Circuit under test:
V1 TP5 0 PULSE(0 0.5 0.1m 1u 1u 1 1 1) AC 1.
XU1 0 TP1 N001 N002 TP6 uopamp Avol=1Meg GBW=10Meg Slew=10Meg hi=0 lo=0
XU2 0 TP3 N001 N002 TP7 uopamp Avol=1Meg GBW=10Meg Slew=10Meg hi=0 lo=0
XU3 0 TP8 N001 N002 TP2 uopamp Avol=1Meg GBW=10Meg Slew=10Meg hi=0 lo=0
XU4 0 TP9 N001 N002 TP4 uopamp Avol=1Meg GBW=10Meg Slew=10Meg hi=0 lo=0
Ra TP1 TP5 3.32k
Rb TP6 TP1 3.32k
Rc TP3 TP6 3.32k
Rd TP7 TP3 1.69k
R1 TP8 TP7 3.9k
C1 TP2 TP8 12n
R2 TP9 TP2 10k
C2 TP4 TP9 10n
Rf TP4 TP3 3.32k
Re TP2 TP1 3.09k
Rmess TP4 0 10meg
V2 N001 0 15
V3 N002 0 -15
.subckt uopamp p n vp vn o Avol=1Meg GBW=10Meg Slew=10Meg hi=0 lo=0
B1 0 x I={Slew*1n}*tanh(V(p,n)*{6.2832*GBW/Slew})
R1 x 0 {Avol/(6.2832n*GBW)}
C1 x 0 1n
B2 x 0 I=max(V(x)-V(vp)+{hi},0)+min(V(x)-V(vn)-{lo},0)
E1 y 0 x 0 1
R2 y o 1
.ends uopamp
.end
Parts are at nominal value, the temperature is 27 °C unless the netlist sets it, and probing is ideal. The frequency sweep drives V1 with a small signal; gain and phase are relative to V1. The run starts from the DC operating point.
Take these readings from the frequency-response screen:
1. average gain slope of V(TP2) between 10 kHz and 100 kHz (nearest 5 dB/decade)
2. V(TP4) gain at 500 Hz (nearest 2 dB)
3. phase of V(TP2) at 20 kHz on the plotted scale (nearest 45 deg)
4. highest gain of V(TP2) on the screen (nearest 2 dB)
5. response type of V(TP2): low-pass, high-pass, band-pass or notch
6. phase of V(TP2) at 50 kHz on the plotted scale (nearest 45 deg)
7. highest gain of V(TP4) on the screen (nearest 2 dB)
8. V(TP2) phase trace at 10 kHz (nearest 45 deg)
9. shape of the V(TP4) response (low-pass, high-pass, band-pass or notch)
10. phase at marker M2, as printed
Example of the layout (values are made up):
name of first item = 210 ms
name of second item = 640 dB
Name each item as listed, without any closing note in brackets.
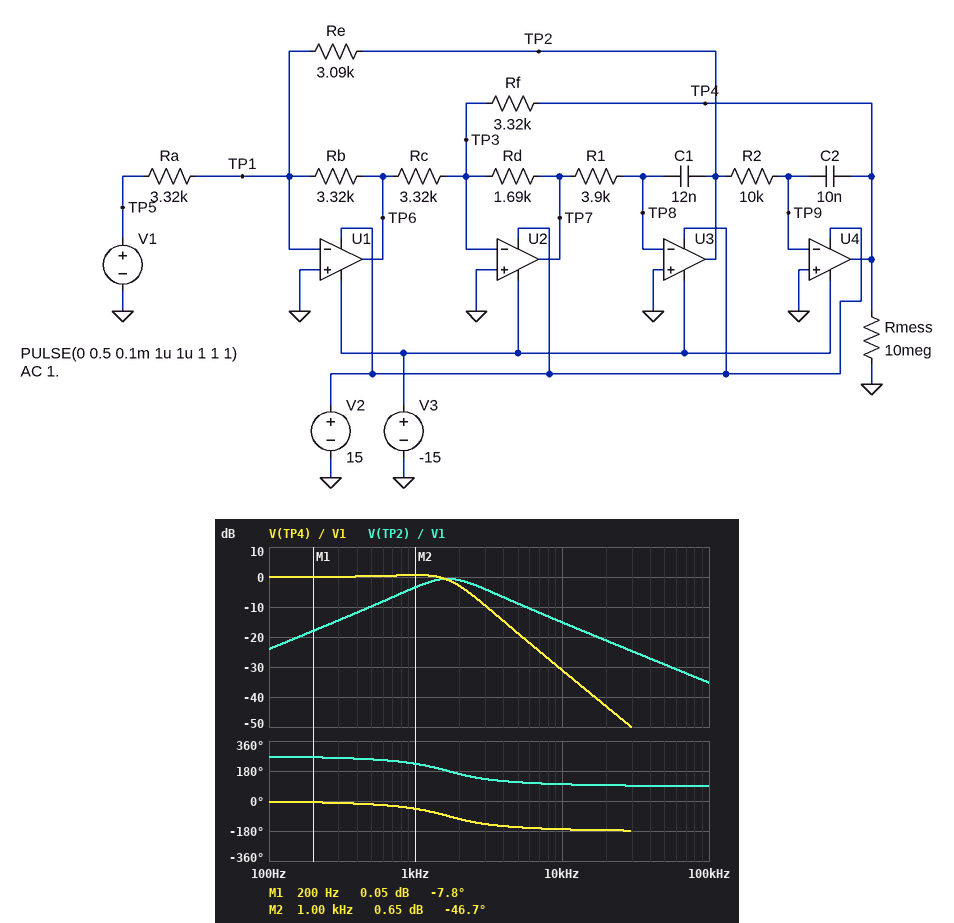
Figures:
average gain slope of V(TP2) between 10 kHz and 100 kHz = -20 dB/decade
V(TP4) gain at 500 Hz = 0 dB
phase of V(TP2) at 20 kHz on the plotted scale = 90 deg
highest gain of V(TP2) on the screen = 0 dB
response type of V(TP2): low-pass, high-pass, band-pass or notch = band-pass
phase of V(TP2) at 50 kHz on the plotted scale = 90 deg
highest gain of V(TP4) on the screen = 0 dB
V(TP2) phase trace at 10 kHz = 90 deg
shape of the V(TP4) response = low-pass
phase at marker M2, as printed = -46.7 deg
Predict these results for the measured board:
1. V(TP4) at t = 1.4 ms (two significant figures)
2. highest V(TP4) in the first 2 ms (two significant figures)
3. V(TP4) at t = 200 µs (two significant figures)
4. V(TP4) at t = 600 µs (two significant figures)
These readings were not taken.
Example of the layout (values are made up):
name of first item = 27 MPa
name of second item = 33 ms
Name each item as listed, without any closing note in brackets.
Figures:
V(TP4) at t = 1.4 ms = 500 mV
highest V(TP4) in the first 2 ms = 560 mV
V(TP4) at t = 200 µs = 170 mV
V(TP4) at t = 600 µs = 530 mV
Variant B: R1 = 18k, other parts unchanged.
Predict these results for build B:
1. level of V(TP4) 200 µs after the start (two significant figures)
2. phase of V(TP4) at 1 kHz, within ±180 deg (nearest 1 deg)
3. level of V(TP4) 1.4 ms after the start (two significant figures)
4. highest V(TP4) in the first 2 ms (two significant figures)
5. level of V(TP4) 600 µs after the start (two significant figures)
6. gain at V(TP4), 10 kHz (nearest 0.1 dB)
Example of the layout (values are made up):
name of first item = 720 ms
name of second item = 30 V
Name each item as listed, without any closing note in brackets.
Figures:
level of V(TP4) 200 µs after the start = 53 mV
phase of V(TP4) at 1 kHz, within ±180 deg = -135 deg
level of V(TP4) 1.4 ms after the start = 410 mV
highest V(TP4) in the first 2 ms = 710 mV
level of V(TP4) 600 µs after the start = 630 mV
gain at V(TP4), 10 kHz = -44.4 dB
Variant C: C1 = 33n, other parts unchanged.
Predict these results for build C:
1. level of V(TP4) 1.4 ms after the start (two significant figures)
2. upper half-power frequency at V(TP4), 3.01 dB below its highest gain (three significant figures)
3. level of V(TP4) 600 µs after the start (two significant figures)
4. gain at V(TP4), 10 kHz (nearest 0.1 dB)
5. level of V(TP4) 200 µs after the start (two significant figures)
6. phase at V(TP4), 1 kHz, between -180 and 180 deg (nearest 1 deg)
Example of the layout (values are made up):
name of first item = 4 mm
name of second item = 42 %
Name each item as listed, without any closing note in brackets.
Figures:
level of V(TP4) 1.4 ms after the start = 480 mV
upper half-power frequency at V(TP4), 3.01 dB below its highest gain = 1.19 kHz
level of V(TP4) 600 µs after the start = 660 mV
gain at V(TP4), 10 kHz = -39.9 dB
level of V(TP4) 200 µs after the start = 83 mV
phase at V(TP4), 1 kHz, between -180 and 180 deg = -90 deg
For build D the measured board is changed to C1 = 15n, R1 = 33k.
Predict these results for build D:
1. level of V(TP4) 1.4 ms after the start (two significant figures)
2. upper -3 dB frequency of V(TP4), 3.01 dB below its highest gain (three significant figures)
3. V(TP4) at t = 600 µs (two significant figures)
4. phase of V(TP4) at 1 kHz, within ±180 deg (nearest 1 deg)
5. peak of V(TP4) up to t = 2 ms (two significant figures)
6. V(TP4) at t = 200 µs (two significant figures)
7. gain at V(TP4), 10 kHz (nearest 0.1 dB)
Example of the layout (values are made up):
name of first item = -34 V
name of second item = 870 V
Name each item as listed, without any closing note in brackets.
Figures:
level of V(TP4) 1.4 ms after the start = 670 mV
upper -3 dB frequency of V(TP4), 3.01 dB below its highest gain = 577 Hz
V(TP4) at t = 600 µs = 440 mV
phase of V(TP4) at 1 kHz, within ±180 deg = -167 deg
peak of V(TP4) up to t = 2 ms = 790 mV
V(TP4) at t = 200 µs = 24 mV
gain at V(TP4), 10 kHz = -51.7 dB
